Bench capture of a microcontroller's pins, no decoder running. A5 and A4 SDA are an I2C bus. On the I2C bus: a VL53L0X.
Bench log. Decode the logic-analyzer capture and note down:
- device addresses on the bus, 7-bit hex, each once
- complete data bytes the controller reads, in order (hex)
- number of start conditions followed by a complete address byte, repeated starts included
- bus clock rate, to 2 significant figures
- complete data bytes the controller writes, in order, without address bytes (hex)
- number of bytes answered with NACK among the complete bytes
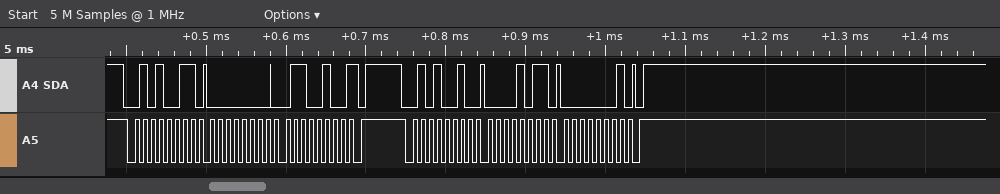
0x29
00 64
2
100 kHz
0B 01
1
